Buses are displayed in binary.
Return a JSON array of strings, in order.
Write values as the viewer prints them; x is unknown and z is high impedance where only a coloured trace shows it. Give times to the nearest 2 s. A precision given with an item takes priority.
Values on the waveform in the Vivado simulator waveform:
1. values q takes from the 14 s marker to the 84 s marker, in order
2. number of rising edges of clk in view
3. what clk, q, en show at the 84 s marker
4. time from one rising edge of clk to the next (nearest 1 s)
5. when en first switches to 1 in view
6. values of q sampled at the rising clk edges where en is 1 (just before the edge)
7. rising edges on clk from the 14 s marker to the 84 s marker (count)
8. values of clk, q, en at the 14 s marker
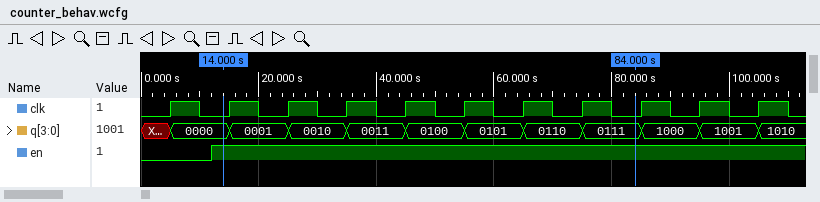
["0000, 0001, 0010, 0011, 0100, 0101, 0110, 0111", "11", "clk=0, q=0111, en=1", "10 s", "12 s", "0000, 0001, 0010, 0011, 0100, 0101, 0110, 0111, 1000, 1001", "7", "clk=0, q=0000, en=1"]
